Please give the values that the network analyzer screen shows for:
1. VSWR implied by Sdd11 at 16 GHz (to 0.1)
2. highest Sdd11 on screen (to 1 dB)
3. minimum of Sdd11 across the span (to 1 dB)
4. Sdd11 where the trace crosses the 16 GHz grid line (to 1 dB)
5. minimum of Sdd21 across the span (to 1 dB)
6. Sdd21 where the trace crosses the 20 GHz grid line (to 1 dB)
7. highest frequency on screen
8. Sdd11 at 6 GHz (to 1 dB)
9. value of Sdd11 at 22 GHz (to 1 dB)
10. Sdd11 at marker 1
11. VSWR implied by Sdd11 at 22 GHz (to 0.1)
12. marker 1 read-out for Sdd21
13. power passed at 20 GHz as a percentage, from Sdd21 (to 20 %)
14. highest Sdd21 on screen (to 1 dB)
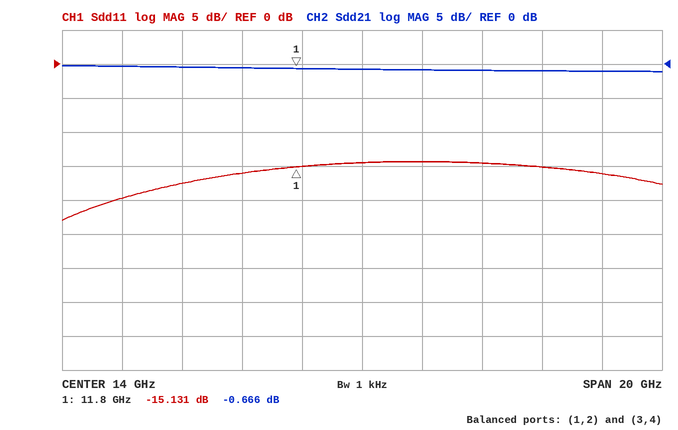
1.5
-14 dB
-23 dB
-14 dB
-1 dB
-1 dB
24 GHz
-20 dB
-16 dB
-15.131 dB
1.4
-0.666 dB
80 %
0 dB
